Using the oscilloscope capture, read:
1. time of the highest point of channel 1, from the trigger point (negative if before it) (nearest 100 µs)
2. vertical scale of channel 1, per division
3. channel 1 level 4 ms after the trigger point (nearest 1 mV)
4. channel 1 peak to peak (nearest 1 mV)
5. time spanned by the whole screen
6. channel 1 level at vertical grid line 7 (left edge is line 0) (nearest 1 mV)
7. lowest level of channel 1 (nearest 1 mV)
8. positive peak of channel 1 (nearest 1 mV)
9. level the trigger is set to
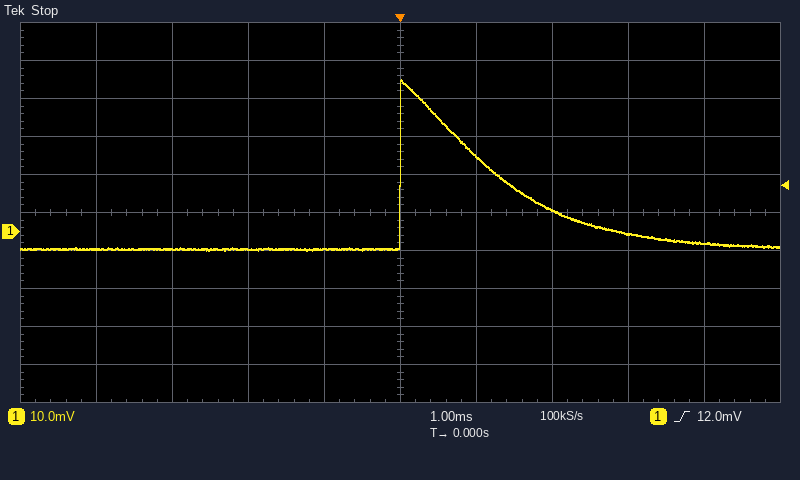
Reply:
0.0 ms
10 mV
-3 mV
45 mV
10 ms
6 mV
-5 mV
40 mV
12.0 mV
